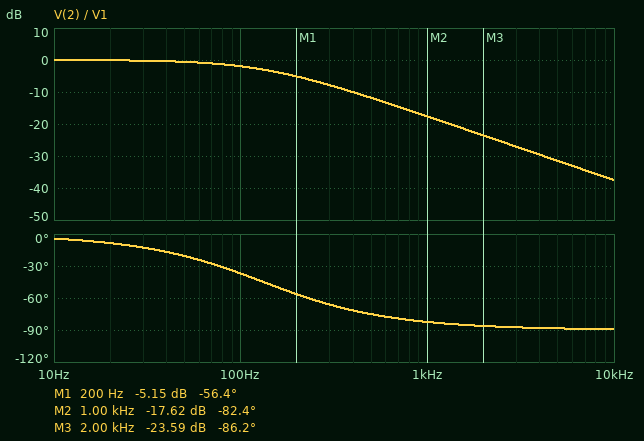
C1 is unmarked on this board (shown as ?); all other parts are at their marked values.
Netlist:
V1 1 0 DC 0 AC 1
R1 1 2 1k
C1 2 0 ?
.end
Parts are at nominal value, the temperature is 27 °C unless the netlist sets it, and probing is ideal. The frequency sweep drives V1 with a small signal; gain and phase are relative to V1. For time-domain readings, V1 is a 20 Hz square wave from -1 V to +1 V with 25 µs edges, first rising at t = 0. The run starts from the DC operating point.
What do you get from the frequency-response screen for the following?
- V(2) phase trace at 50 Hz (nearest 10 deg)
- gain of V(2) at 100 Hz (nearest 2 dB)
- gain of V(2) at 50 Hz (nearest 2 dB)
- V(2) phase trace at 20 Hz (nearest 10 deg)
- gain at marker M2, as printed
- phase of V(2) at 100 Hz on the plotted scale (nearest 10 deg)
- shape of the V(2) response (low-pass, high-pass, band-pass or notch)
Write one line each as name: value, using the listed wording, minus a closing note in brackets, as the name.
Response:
V(2) phase trace at 50 Hz: -20 deg
gain of V(2) at 100 Hz: -2 dB
gain of V(2) at 50 Hz: 0 dB
V(2) phase trace at 20 Hz: -10 deg
gain at marker M2, as printed: -17.62 dB
phase of V(2) at 100 Hz on the plotted scale: -40 deg
shape of the V(2) response: low-pass
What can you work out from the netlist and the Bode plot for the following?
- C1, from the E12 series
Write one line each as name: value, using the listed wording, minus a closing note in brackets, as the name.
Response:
C1, from the E12 series: 1.2 µF
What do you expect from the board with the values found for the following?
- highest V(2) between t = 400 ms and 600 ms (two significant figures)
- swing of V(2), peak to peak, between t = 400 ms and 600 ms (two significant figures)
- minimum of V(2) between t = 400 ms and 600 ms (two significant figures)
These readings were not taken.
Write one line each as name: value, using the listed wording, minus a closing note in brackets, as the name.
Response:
highest V(2) between t = 400 ms and 600 ms: 1.0 V
swing of V(2), peak to peak, between t = 400 ms and 600 ms: 2.0 V
minimum of V(2) between t = 400 ms and 600 ms: -1.0 V
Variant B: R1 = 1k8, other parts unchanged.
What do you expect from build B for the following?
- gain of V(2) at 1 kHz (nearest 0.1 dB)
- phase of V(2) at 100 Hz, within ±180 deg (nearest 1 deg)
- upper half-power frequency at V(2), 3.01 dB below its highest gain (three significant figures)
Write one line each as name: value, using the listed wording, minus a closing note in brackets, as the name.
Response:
gain of V(2) at 1 kHz: -22.7 dB
phase of V(2) at 100 Hz, within ±180 deg: -54 deg
upper half-power frequency at V(2), 3.01 dB below its highest gain: 73.7 Hz
